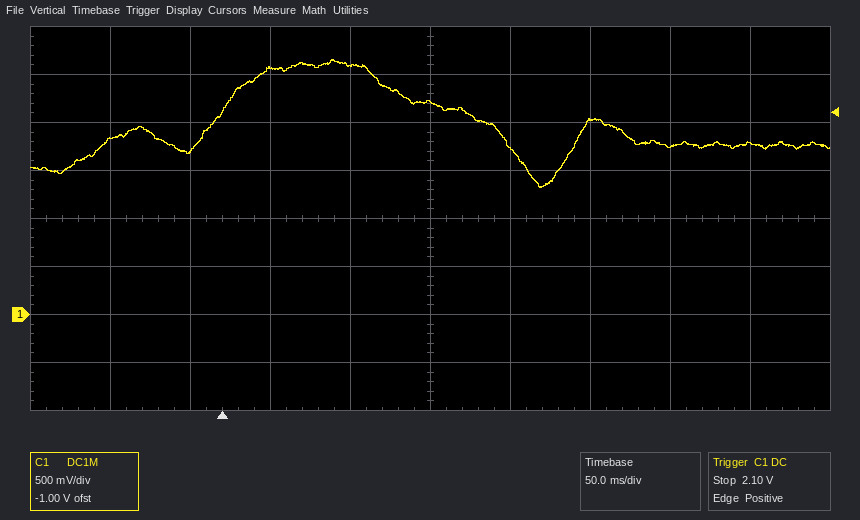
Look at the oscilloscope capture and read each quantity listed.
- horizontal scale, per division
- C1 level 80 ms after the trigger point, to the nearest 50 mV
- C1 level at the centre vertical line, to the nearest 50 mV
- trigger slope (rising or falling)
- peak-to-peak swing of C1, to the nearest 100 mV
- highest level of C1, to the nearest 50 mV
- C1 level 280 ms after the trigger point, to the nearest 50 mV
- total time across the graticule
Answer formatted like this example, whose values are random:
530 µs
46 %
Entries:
50 ms
2.60 V
2.20 V
rising
1.30 V
2.65 V
1.75 V
500 ms
